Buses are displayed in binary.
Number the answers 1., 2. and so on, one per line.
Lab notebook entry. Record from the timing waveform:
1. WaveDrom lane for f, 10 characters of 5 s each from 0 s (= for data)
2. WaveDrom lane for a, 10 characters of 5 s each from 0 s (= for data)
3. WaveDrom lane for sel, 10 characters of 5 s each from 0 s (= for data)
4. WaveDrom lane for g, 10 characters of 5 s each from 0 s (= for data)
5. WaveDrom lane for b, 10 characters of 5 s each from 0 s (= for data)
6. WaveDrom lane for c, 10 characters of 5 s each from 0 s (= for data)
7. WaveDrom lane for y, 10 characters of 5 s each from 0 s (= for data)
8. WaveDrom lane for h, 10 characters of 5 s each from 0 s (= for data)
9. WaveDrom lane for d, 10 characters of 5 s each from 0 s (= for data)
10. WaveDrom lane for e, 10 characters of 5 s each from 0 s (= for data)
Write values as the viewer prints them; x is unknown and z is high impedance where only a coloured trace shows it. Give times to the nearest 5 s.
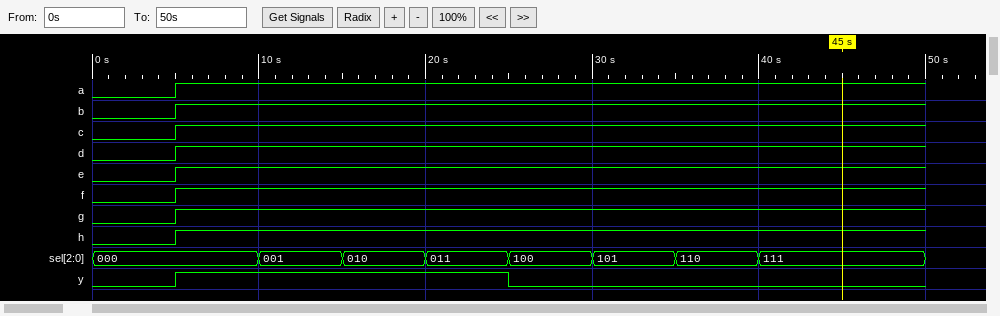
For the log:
1. {name: 'f', wave: '01........'}
2. {name: 'a', wave: '01........'}
3. {name: 'sel', wave: '=.=======.', data: '000 001 010 011 100 101 110 111'}
4. {name: 'g', wave: '01........'}
5. {name: 'b', wave: '01........'}
6. {name: 'c', wave: '01........'}
7. {name: 'y', wave: '01...0....'}
8. {name: 'h', wave: '01........'}
9. {name: 'd', wave: '01........'}
10. {name: 'e', wave: '01........'}
